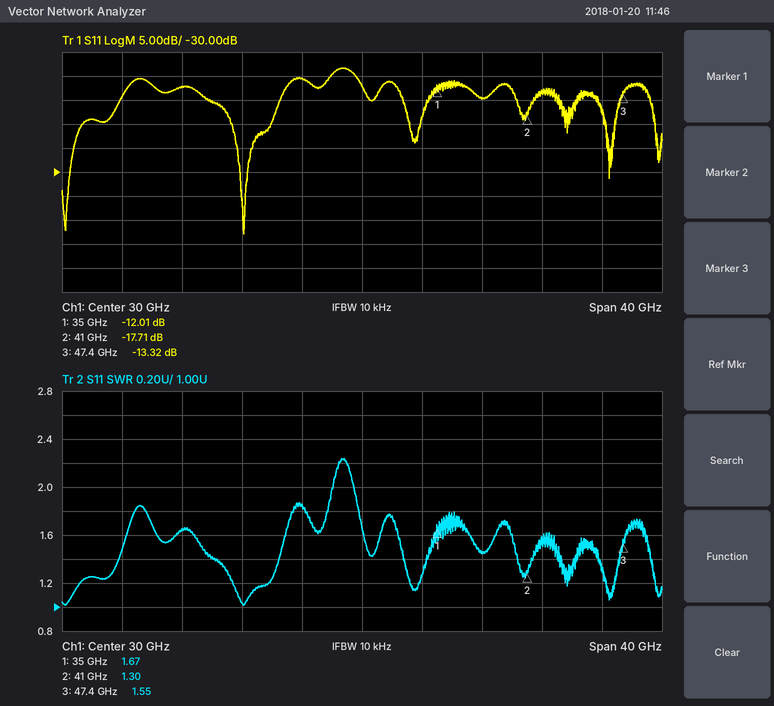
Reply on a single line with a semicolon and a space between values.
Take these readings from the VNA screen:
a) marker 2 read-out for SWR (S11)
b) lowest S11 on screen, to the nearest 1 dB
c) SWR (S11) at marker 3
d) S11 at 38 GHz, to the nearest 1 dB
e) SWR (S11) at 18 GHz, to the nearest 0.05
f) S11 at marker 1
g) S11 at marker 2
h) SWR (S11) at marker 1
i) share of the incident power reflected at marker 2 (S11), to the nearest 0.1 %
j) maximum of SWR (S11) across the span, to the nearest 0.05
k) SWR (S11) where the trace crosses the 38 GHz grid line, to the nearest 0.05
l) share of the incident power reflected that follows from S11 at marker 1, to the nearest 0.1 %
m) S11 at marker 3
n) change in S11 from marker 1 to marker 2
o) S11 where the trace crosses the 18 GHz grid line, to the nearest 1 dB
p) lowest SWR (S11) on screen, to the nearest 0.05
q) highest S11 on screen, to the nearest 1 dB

1.30; -43 dB; 1.55; -15 dB; 1.65; -12.01 dB; -17.71 dB; 1.67; 1.7 %; 2.25; 1.45; 6.3 %; -13.32 dB; -5.70 dB; -12 dB; 1.00; -8 dB
